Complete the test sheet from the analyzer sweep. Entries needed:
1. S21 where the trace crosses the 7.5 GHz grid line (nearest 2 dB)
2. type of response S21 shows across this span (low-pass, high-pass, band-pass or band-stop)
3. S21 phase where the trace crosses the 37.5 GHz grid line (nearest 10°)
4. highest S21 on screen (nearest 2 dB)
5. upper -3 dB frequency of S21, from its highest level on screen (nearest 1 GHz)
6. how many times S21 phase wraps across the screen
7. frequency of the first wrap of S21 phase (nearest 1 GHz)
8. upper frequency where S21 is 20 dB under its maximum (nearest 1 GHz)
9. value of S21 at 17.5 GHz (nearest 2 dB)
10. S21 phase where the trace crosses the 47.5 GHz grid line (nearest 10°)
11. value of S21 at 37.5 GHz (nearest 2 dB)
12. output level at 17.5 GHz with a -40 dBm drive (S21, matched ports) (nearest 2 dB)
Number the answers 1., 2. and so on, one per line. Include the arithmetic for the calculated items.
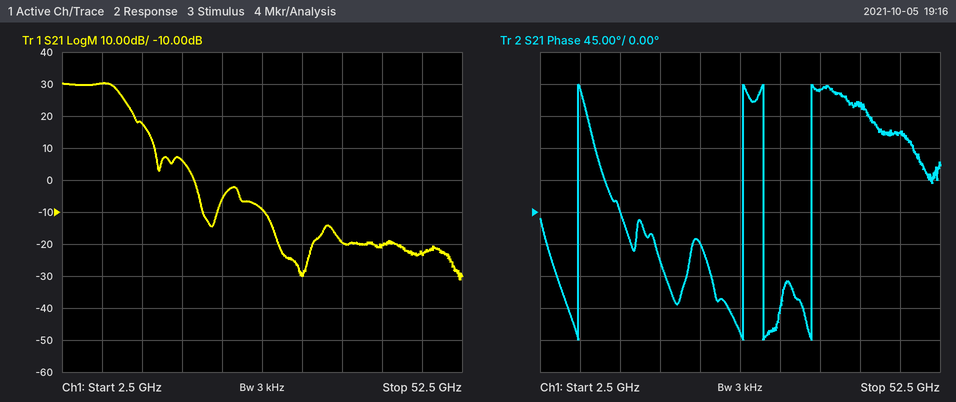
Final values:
1. 30 dB
2. low-pass
3. 170°
4. 30 dB
5. 10 GHz
6. 4
7. 7 GHz
8. 14 GHz
9. 6 dB
10. 110°
11. -20 dB
12. -40 dBm + (6 dB) = -34 dBm
